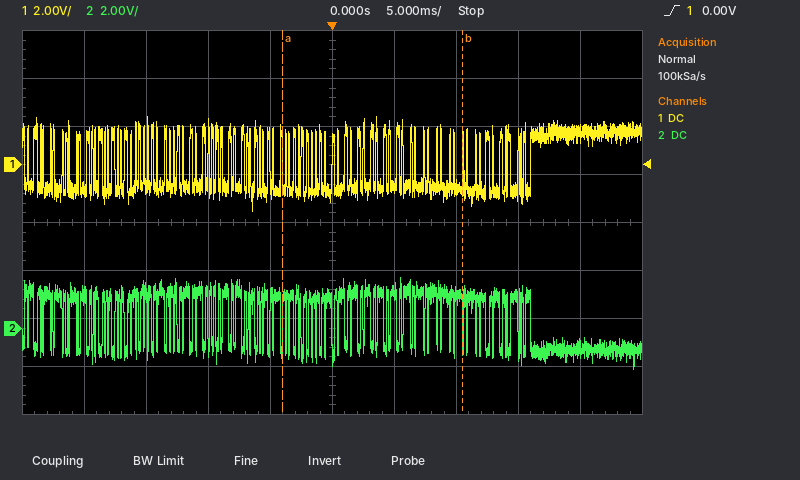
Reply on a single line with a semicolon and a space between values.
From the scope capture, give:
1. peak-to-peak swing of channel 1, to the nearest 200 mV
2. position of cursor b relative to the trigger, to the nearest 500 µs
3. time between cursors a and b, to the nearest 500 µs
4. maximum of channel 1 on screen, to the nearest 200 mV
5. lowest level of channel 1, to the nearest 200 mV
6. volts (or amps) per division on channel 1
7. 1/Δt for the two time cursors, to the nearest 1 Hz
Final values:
4.0 V; +10.5 ms; 14.5 ms; 2.0 V; -2.0 V; 2 V; 69 Hz
